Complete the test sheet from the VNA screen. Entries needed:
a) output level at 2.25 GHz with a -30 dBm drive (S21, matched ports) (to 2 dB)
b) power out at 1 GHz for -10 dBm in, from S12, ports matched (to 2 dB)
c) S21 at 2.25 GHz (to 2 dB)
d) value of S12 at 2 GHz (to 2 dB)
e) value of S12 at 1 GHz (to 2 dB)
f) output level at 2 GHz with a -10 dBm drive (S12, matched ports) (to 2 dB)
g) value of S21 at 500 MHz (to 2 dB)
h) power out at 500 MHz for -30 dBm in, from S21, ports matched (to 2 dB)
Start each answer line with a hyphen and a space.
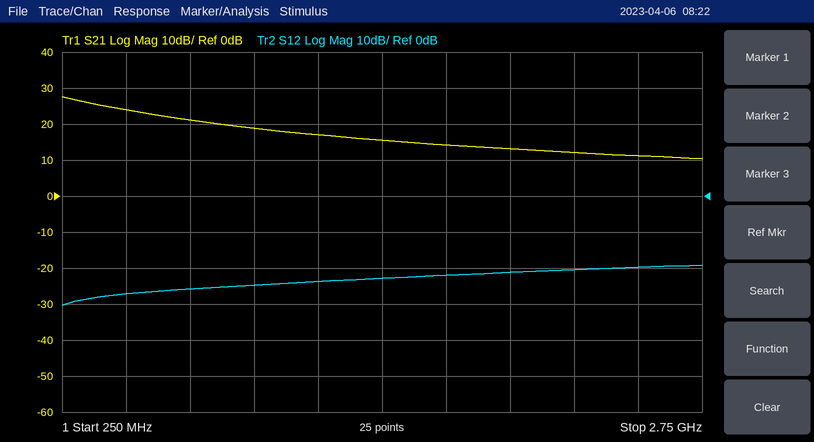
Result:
- -18 dBm
- -34 dBm
- 12 dB
- -22 dB
- -24 dB
- -32 dBm
- 24 dB
- -6 dBm
